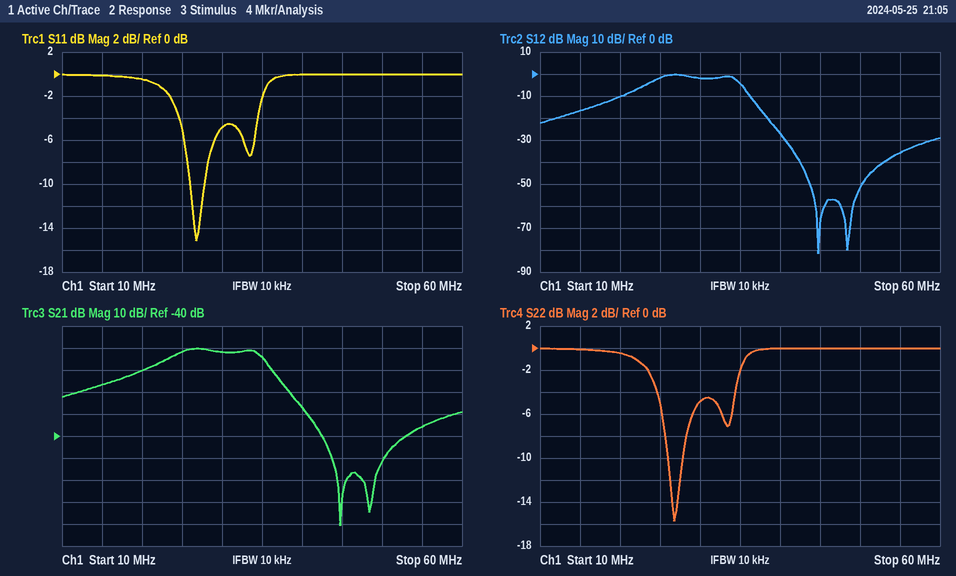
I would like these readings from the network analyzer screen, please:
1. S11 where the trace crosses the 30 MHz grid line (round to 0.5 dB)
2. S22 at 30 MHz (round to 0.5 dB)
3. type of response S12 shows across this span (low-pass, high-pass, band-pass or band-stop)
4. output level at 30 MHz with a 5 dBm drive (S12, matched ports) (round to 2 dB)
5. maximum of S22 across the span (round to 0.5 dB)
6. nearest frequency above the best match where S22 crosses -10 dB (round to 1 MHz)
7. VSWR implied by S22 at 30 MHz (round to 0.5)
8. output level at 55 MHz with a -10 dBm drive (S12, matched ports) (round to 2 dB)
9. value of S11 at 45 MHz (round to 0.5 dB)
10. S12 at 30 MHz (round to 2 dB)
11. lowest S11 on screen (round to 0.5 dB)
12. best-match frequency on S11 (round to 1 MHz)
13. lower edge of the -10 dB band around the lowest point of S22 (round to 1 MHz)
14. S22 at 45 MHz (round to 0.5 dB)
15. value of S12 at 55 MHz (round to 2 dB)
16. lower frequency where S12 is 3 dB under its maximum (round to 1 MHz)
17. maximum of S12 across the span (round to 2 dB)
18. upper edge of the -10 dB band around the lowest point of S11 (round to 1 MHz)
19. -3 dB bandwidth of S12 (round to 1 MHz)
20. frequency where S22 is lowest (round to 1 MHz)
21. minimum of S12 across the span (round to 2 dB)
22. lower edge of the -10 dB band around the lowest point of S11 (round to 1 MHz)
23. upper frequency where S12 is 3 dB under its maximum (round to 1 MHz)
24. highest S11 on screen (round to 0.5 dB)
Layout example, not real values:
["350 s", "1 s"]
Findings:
["-5.0 dB", "-5.0 dB", "band-pass", "4 dBm", "0.0 dB", "28 MHz", "3.5", "-46 dBm", "0.0 dB", "-2 dB", "-15.0 dB", "27 MHz", "26 MHz", "0.0 dB", "-36 dB", "24 MHz", "0 dB", "28 MHz", "11 MHz", "27 MHz", "-82 dB", "26 MHz", "35 MHz", "0.0 dB"]
